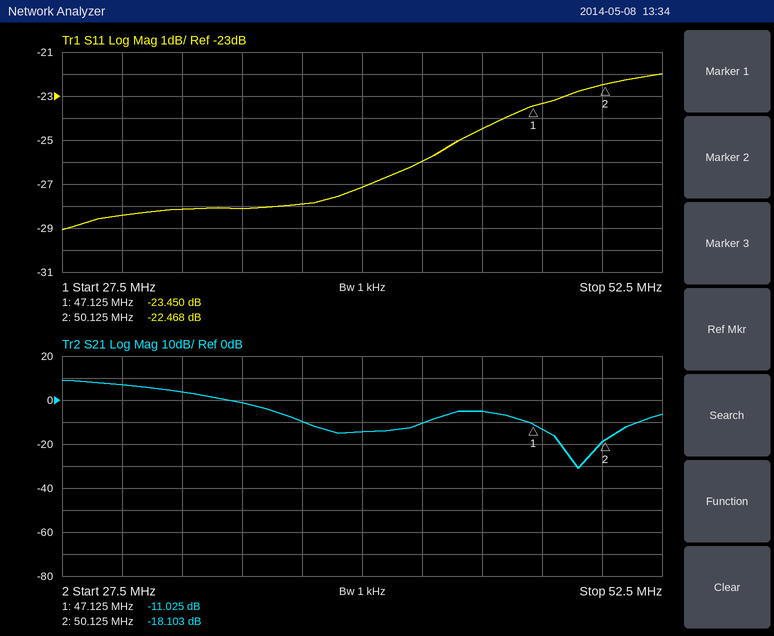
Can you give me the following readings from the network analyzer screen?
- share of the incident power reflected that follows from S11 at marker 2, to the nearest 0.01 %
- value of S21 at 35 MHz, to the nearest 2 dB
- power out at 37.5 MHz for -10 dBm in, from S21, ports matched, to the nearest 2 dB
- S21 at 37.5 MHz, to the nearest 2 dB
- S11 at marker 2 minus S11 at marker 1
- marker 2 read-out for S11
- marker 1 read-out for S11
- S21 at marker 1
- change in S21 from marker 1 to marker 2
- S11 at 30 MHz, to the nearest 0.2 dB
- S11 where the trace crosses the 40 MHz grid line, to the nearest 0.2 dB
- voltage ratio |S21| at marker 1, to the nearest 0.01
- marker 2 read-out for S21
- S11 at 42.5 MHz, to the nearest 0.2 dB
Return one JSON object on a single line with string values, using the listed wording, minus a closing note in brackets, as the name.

{"share of the incident power reflected that follows from S11 at marker 2, to the nearest 0.01 %": "0.57 %", "value of S21 at 35 MHz, to the nearest 2 dB": "-2 dB", "power out at 37.5 MHz for -10 dBm in, from S21, ports matched, to the nearest 2 dB": "-20 dBm", "S21 at 37.5 MHz, to the nearest 2 dB": "-10 dB", "S11 at marker 2 minus S11 at marker 1": "0.982 dB", "marker 2 read-out for S11": "-22.468 dB", "marker 1 read-out for S11": "-23.450 dB", "S21 at marker 1": "-11.025 dB", "change in S21 from marker 1 to marker 2": "-7.078 dB", "S11 at 30 MHz, to the nearest 0.2 dB": "-28.4 dB", "S11 where the trace crosses the 40 MHz grid line, to the nearest 0.2 dB": "-27.2 dB", "voltage ratio |S21| at marker 1, to the nearest 0.01": "0.28", "marker 2 read-out for S21": "-18.103 dB", "S11 at 42.5 MHz, to the nearest 0.2 dB": "-26.0 dB"}
